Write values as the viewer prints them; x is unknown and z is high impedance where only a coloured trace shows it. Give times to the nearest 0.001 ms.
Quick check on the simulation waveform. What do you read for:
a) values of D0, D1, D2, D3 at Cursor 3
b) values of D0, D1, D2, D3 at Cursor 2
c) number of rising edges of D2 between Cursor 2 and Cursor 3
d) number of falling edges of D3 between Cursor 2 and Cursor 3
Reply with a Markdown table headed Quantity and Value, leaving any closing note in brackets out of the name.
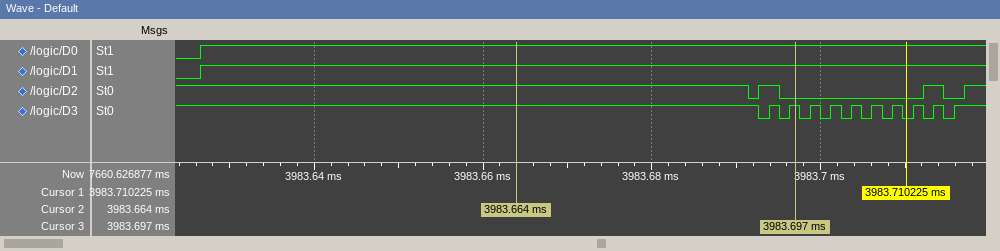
| Quantity | Value |
|---|---|
| values of D0, D1, D2, D3 at Cursor 3 | D0=1, D1=1, D2=0, D3=1 |
| values of D0, D1, D2, D3 at Cursor 2 | D0=1, D1=1, D2=1, D3=1 |
| number of rising edges of D2 between Cursor 2 and Cursor 3 | 1 |
| number of falling edges of D3 between Cursor 2 and Cursor 3 | 2 |
